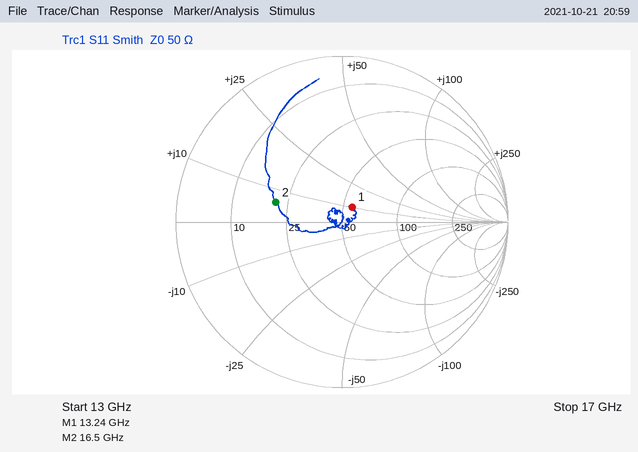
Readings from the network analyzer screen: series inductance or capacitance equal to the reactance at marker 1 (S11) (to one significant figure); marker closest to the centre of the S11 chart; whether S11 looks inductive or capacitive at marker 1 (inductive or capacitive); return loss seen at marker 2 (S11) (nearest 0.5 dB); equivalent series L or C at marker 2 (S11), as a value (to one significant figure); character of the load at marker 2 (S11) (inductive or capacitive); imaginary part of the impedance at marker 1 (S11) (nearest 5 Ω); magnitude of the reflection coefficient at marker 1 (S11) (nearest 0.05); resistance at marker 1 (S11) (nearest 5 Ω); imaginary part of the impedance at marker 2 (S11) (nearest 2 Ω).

100 pH
marker 1
inductive
7.5 dB
60 pH
inductive
+10 Ω
0.10
55 Ω
+6 Ω
